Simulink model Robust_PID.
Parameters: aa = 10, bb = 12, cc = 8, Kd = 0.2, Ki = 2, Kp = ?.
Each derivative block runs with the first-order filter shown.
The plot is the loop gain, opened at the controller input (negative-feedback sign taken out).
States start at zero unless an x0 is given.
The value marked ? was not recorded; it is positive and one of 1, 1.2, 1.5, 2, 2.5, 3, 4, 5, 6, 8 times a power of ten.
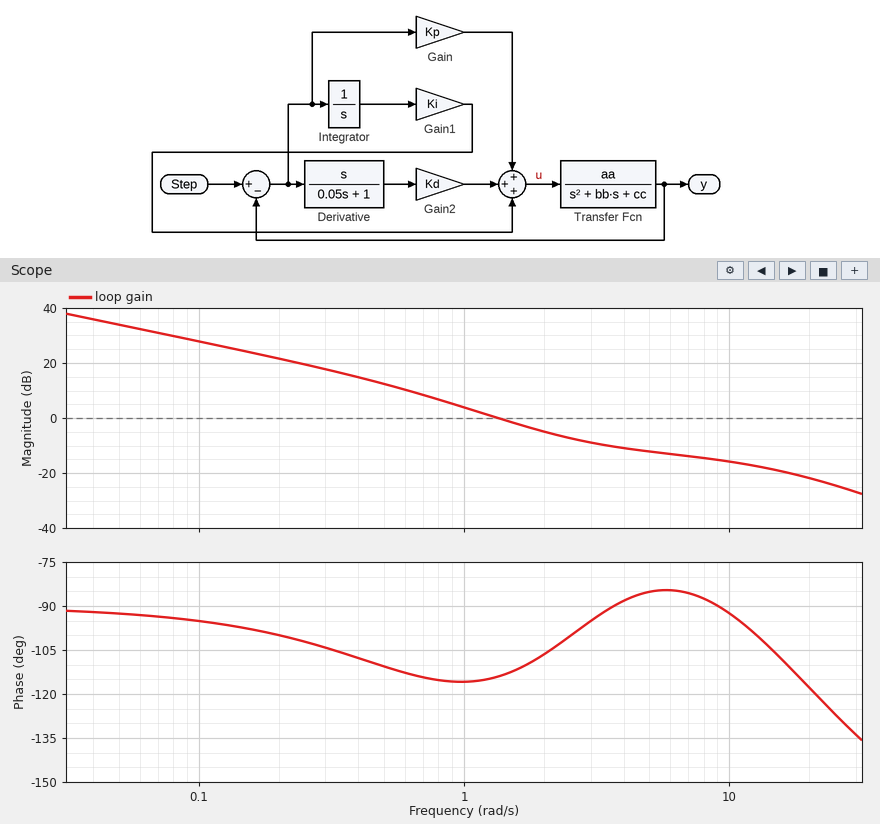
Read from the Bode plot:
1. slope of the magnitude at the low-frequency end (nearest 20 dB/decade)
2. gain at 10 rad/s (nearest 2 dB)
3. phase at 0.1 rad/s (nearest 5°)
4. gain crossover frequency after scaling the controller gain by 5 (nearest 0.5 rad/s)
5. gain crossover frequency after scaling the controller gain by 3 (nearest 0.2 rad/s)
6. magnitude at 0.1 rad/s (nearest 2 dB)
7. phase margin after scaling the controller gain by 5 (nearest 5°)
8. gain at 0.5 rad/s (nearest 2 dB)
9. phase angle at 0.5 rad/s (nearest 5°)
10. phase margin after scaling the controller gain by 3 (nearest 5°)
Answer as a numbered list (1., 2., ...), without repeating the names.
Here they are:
1. -20 dB/decade
2. -16 dB
3. -95°
4. 7.0 rad/s
5. 3.2 rad/s
6. 28 dB
7. 95°
8. 12 dB
9. -110°
10. 85°
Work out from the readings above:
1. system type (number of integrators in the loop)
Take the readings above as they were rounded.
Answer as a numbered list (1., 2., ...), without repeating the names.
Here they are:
1. 1
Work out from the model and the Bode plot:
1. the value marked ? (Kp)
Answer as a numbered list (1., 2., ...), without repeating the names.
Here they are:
1. 1.2
